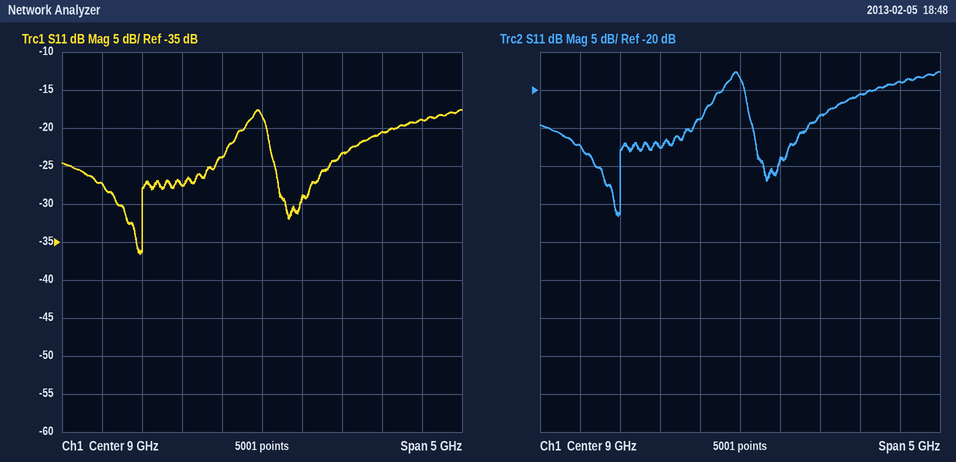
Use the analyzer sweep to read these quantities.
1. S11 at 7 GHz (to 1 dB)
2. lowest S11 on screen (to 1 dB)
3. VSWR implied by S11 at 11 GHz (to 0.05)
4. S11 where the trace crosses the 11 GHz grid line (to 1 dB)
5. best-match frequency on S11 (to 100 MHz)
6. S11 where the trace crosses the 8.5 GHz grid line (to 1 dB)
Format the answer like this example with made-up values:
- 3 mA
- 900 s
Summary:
- -27 dB
- -37 dB
- 1.25
- -19 dB
- 7.5 GHz
- -24 dB
